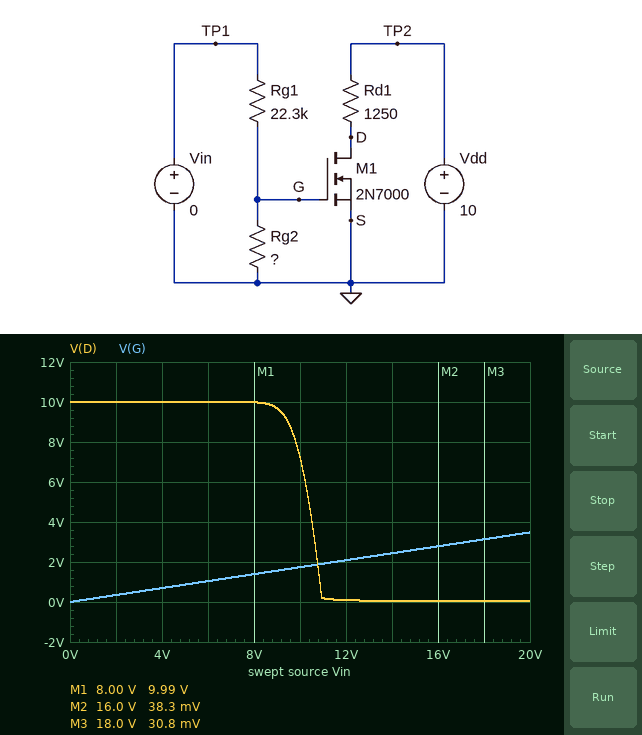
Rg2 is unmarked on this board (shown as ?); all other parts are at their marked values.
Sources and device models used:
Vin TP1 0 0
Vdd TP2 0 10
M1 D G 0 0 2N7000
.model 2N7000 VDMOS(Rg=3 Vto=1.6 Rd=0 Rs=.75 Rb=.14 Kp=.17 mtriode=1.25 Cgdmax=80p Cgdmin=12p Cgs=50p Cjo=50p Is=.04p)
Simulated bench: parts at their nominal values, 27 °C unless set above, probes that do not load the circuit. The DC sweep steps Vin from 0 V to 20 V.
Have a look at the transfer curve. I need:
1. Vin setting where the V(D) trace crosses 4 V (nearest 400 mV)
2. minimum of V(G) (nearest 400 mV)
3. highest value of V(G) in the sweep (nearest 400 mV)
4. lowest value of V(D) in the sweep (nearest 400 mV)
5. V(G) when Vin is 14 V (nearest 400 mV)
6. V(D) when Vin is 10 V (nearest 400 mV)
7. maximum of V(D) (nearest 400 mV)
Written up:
10.4 V
0 V
3.6 V
0 V
2.4 V
7.2 V
10.0 V
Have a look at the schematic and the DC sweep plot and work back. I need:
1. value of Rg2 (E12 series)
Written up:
4.7 kΩ
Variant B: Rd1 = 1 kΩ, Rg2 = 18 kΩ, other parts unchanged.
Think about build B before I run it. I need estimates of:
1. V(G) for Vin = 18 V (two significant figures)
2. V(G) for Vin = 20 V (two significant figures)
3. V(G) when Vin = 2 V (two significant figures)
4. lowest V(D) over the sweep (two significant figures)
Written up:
8.0 V
8.9 V
890 mV
14 mV
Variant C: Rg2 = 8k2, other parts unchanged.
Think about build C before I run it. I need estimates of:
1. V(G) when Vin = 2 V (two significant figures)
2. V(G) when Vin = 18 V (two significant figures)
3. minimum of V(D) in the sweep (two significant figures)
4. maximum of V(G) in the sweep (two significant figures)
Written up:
540 mV
4.8 V
16 mV
5.4 V
